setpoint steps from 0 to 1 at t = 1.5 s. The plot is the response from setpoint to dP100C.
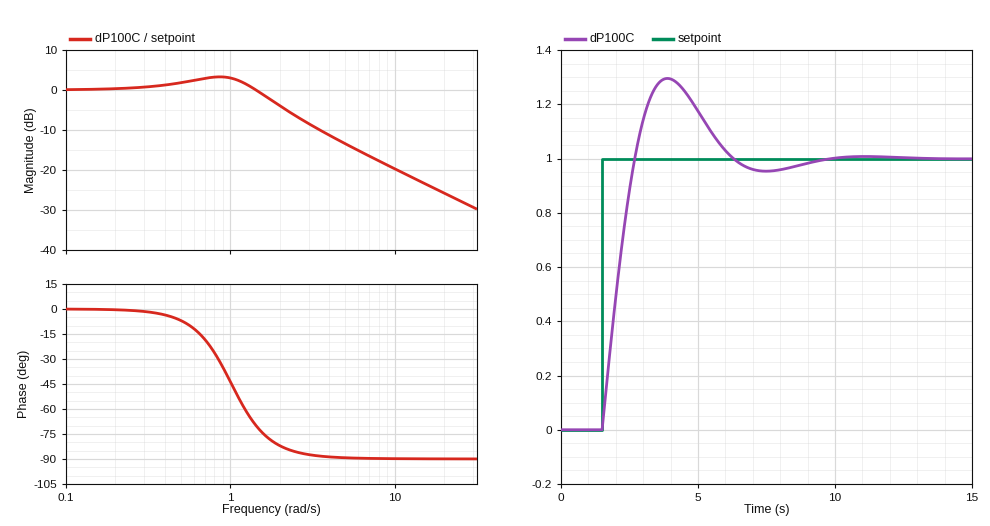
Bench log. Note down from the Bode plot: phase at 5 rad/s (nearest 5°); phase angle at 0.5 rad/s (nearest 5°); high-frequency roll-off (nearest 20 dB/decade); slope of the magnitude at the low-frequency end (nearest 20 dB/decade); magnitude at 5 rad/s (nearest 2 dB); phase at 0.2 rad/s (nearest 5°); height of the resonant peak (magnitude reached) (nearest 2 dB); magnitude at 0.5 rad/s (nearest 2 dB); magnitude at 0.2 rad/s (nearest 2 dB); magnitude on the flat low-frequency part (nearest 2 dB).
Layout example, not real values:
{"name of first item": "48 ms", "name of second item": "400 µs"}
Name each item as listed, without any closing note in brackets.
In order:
{"phase at 5 rad/s": "-90°", "phase angle at 0.5 rad/s": "-5°", "high-frequency roll-off": "-20 dB/decade", "slope of the magnitude at the low-frequency end": "0 dB/decade", "magnitude at 5 rad/s": "-14 dB", "phase at 0.2 rad/s": "0°", "height of the resonant peak (magnitude reached)": "4 dB", "magnitude at 0.5 rad/s": "2 dB", "magnitude at 0.2 rad/s": "0 dB", "magnitude on the flat low-frequency part": "0 dB"}
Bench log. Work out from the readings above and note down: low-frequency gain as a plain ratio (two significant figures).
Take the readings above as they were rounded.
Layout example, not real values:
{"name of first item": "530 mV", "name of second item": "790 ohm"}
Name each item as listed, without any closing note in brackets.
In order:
{"low-frequency gain as a plain ratio": "1.0"}
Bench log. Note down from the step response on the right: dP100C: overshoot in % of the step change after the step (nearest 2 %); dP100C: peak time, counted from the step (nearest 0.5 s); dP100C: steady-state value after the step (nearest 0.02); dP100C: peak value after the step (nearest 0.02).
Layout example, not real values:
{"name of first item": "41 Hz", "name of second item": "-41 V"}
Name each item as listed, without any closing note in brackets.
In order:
{"dP100C: overshoot in % of the step change after the step": "30 %", "dP100C: peak time, counted from the step": "2.5 s", "dP100C: steady-state value after the step": "1.00", "dP100C: peak value after the step": "1.30"}
